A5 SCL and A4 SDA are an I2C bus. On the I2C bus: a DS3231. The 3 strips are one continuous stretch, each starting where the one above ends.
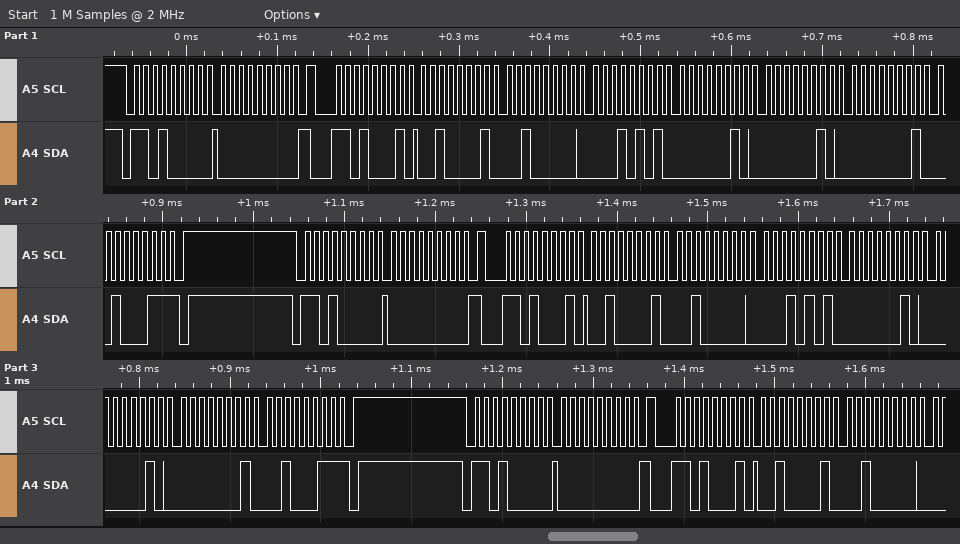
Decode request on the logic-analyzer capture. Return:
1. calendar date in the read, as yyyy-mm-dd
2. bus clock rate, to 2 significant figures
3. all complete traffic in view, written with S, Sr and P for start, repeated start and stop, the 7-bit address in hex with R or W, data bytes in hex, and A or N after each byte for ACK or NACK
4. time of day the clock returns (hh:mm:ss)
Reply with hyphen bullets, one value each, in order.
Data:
- 2023-01-02
- 100 kHz
- S 68W A 00 A Sr 68R A 21 A 20 A 15 A 02 A 02 A 01 A 23 N P S 68W A 00 A Sr 68R A 21 A 20 A 15 A 02 A 02 A 01 A 23 N P S 68W A 00 A Sr 68R A 21 A 20 A
- 15:20:21
